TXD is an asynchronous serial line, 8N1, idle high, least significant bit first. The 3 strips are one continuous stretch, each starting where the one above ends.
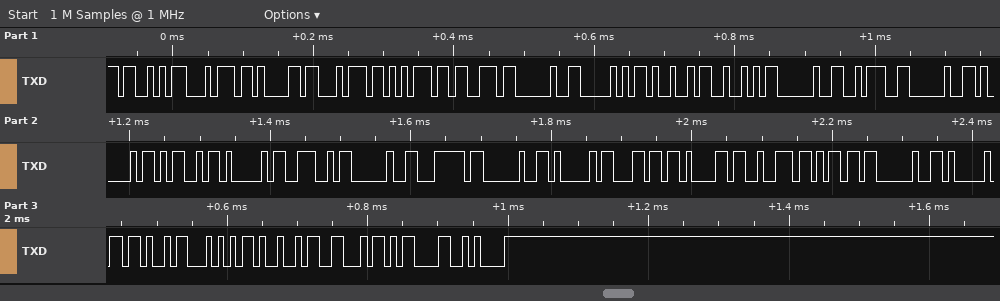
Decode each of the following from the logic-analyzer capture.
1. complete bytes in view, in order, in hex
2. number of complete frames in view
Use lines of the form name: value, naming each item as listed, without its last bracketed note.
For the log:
complete bytes in view, in order, in hex: 53 74 61 74 75 73 20 50 49 52 20 3A 20 41 4D 41 4E 20 7C 20 41 6C 61 72 6D 20 41 4B 54 49 46 0D 0A
number of complete frames in view: 33
